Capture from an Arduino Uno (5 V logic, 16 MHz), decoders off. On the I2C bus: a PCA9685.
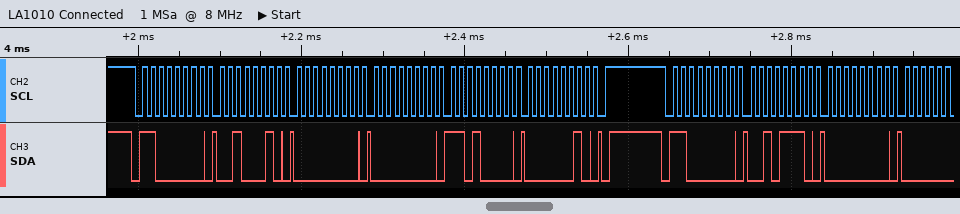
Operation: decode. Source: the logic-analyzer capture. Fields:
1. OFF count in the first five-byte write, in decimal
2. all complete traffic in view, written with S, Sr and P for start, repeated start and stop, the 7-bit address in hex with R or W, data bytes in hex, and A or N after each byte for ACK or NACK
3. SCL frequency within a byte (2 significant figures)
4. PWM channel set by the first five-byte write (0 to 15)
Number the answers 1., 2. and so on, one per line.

1. 720
2. S 60W A 22 A 00 A 00 A D0 A 02 A P S 60W A 2E A 00 A
3. 100 kHz
4. 7
